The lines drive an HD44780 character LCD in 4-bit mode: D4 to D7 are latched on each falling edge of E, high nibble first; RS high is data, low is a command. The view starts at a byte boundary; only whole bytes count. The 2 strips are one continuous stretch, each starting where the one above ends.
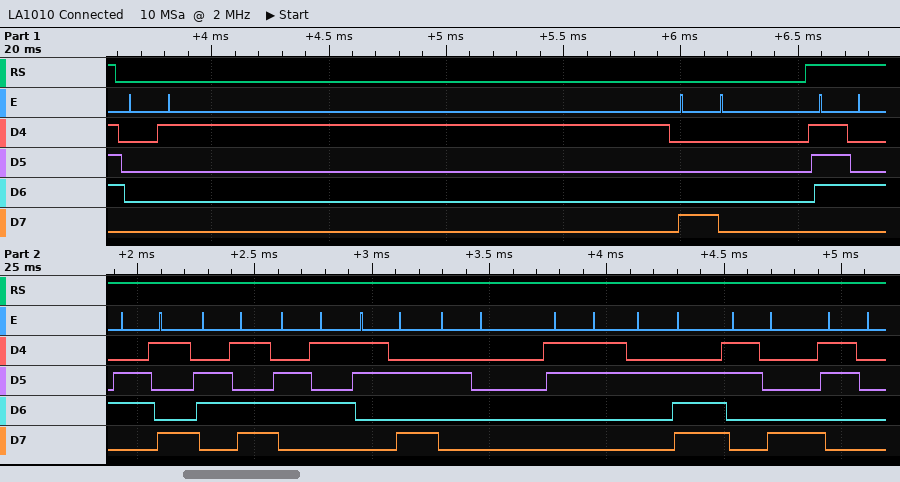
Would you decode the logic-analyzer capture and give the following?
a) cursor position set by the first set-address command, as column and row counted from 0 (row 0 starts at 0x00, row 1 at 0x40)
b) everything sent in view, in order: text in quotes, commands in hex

column 0, row 0
0x01 0x80 "time: 3.80"
